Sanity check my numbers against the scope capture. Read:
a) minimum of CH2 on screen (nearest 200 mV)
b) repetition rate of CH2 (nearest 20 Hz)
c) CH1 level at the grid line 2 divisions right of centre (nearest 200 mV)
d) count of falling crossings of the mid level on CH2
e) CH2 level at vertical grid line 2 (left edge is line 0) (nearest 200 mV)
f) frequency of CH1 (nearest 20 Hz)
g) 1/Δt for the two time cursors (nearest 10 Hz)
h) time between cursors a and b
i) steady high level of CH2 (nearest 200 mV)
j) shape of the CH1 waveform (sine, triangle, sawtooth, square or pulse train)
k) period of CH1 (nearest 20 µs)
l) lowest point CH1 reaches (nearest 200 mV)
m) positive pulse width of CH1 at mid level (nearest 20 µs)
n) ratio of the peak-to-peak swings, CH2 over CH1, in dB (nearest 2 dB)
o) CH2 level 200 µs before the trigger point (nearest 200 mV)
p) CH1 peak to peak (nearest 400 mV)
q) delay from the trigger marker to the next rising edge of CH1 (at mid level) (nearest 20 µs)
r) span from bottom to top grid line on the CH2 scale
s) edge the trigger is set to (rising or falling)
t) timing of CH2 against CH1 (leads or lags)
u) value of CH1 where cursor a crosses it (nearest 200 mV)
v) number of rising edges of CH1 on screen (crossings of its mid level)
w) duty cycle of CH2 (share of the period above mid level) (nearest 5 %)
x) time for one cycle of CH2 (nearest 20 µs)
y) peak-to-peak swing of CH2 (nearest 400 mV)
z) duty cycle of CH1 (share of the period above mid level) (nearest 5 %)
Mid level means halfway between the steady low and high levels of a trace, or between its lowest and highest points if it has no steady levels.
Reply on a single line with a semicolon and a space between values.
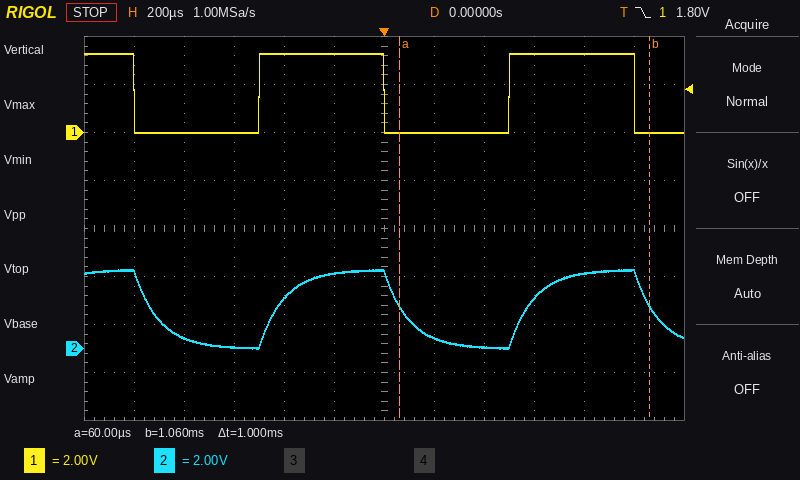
0.0 V; 1.00 kHz; 0.0 V; 3; 400 mV; 1.00 kHz; 1.00 kHz; 1 ms; 3.2 V; square; 1.00 ms; 0.0 V; 500 µs; 0 dB; 3.2 V; 3.2 V; 500 µs; 16 V; falling; lags; 0.0 V; 2; 50 %; 1.00 ms; 3.2 V; 50 %
